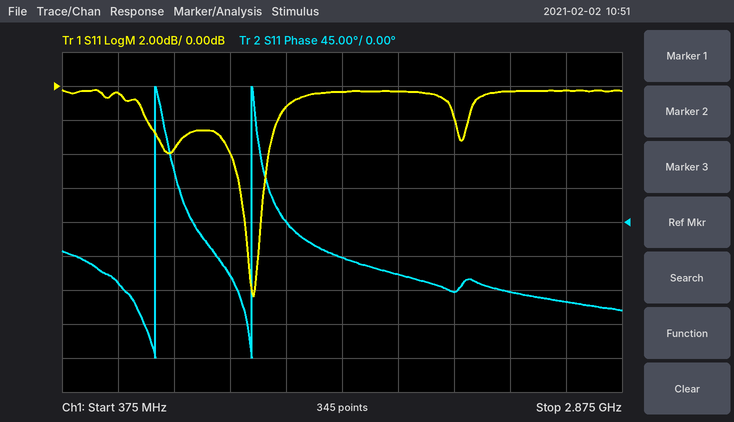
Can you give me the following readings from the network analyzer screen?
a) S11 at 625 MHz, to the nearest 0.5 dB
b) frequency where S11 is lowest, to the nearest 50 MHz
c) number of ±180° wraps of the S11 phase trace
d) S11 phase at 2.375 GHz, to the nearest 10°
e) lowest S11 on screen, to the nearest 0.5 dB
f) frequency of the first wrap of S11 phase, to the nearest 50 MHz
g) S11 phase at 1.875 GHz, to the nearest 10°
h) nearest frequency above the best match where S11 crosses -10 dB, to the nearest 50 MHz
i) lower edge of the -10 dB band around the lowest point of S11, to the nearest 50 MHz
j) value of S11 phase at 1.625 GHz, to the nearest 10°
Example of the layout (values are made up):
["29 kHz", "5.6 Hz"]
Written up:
["-0.5 dB", "1.25 GHz", "2", "-90°", "-12.5 dB", "800 MHz", "-70°", "1.25 GHz", "1.20 GHz", "-50°"]
